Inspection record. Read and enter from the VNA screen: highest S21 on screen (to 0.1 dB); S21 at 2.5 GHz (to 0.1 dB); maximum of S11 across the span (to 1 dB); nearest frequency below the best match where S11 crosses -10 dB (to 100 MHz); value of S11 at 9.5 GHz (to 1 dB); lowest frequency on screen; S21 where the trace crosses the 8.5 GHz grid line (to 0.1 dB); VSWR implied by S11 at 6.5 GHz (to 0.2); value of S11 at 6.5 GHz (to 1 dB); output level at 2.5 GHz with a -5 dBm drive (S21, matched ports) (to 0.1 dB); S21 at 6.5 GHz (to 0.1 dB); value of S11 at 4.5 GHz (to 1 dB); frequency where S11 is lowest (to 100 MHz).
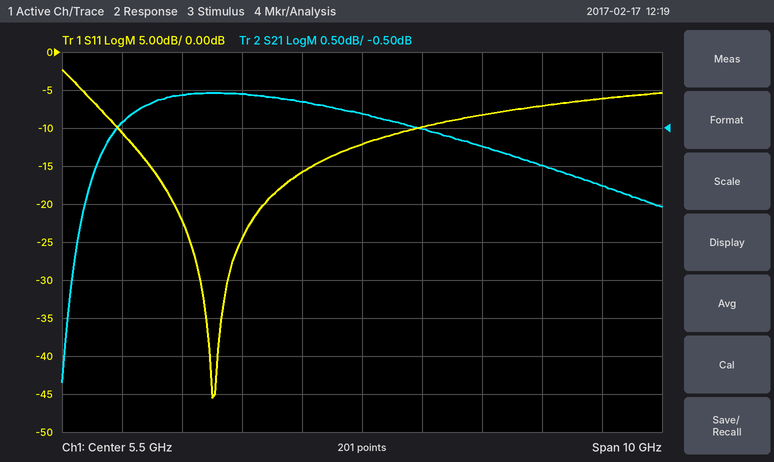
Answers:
0.0 dB
-0.1 dB
-2 dB
1.4 GHz
-6 dB
500 MHz
-1.0 dB
2.0
-10 dB
-5.1 dBm
-0.5 dB
-16 dB
3.0 GHz
